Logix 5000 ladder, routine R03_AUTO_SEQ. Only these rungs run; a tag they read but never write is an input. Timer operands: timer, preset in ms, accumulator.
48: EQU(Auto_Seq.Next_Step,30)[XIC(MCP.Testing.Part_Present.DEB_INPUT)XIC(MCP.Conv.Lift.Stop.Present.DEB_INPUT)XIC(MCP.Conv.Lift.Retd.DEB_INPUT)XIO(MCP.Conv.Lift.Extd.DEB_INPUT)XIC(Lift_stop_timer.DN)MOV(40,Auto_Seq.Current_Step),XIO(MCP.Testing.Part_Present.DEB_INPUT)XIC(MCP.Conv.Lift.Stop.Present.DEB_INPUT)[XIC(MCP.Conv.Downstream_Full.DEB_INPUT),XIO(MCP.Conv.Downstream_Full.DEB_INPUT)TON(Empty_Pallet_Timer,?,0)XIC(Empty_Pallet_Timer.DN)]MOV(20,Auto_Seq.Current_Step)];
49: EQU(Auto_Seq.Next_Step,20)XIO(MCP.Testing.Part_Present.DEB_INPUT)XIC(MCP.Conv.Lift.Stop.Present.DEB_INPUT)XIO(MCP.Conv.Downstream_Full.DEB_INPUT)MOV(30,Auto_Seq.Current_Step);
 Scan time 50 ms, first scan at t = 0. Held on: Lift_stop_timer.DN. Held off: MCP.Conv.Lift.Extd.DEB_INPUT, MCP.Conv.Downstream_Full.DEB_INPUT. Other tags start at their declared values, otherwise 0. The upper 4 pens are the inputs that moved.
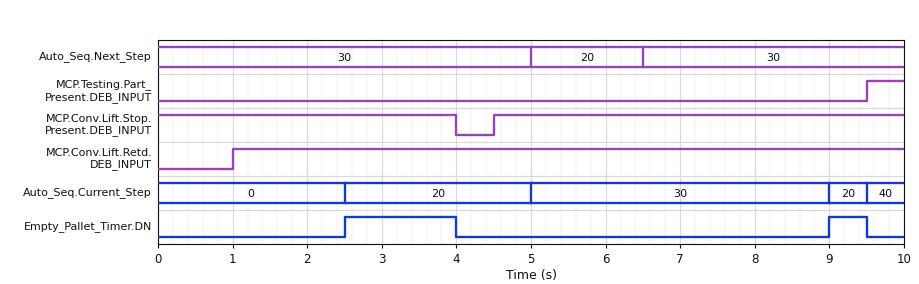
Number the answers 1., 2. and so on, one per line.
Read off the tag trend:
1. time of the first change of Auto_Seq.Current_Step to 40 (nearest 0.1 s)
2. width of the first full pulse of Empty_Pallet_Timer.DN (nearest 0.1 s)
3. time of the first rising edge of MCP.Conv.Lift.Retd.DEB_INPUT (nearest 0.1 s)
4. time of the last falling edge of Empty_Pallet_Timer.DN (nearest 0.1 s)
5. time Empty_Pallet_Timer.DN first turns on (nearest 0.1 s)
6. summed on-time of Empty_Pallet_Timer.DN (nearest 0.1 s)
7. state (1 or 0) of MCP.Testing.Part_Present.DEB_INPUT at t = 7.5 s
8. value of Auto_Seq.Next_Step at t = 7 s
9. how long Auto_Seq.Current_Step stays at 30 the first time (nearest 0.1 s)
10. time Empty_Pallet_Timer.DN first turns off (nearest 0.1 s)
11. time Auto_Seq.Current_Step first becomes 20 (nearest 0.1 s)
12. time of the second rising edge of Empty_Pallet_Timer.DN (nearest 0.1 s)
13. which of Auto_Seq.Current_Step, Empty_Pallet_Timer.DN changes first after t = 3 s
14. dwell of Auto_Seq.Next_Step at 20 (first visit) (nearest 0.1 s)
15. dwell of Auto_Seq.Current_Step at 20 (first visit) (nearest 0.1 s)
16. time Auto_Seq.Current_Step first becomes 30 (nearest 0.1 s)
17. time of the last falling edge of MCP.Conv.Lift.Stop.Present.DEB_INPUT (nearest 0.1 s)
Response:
1. 9.5 s
2. 1.5 s
3. 1.0 s
4. 9.5 s
5. 2.5 s
6. 2.0 s
7. 0
8. 30
9. 4.0 s
10. 4.0 s
11. 2.5 s
12. 9.0 s
13. Empty_Pallet_Timer.DN
14. 1.5 s
15. 2.5 s
16. 5.0 s
17. 4.0 s
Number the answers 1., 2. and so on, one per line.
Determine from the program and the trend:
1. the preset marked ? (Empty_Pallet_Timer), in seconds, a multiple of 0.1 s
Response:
1. 2.5 s
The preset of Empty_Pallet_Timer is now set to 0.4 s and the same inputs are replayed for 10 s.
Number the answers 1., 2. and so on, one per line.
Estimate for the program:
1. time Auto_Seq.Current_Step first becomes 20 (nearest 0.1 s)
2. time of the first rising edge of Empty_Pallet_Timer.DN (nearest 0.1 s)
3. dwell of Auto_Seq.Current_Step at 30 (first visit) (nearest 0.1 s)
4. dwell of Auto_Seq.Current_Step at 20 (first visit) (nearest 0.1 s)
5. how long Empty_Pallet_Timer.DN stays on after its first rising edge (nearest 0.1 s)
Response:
1. 0.4 s
2. 0.4 s
3. 1.9 s
4. 4.6 s
5. 3.6 s
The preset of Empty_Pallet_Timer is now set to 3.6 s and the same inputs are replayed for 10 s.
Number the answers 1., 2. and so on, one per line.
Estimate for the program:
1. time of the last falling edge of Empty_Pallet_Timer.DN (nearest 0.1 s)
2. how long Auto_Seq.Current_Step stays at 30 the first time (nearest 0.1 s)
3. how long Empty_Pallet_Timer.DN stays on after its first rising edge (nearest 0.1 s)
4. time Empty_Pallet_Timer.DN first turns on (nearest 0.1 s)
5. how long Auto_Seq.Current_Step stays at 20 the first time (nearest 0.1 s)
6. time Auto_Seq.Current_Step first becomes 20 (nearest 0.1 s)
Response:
1. 4.0 s
2. 4.5 s
3. 0.4 s
4. 3.6 s
5. 1.4 s
6. 3.6 s
